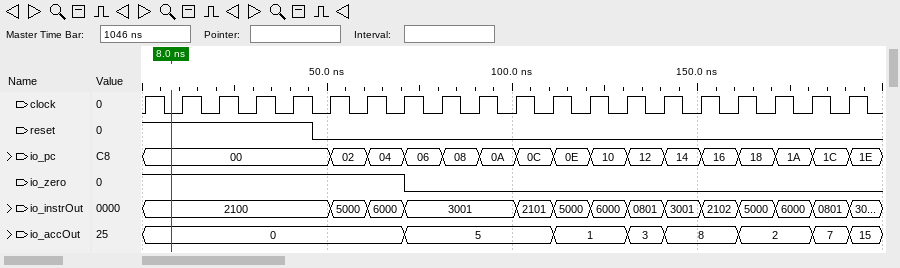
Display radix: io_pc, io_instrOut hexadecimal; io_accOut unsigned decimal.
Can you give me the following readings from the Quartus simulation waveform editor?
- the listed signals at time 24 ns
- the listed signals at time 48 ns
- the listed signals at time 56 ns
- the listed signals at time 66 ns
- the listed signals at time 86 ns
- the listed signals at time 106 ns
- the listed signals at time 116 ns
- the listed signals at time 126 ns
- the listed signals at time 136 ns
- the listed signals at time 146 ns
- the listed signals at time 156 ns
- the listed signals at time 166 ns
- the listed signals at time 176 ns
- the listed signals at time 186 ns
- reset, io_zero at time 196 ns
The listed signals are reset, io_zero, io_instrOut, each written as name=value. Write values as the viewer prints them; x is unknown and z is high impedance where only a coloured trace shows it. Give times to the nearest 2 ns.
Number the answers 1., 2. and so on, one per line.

1. reset=1, io_zero=1, io_instrOut=2100
2. reset=0, io_zero=1, io_instrOut=2100
3. reset=0, io_zero=1, io_instrOut=5000
4. reset=0, io_zero=1, io_instrOut=6000
5. reset=0, io_zero=0, io_instrOut=3001
6. reset=0, io_zero=0, io_instrOut=2101
7. reset=0, io_zero=0, io_instrOut=5000
8. reset=0, io_zero=0, io_instrOut=6000
9. reset=0, io_zero=0, io_instrOut=0801
10. reset=0, io_zero=0, io_instrOut=3001
11. reset=0, io_zero=0, io_instrOut=2102
12. reset=0, io_zero=0, io_instrOut=5000
13. reset=0, io_zero=0, io_instrOut=6000
14. reset=0, io_zero=0, io_instrOut=0801
15. reset=0, io_zero=0
